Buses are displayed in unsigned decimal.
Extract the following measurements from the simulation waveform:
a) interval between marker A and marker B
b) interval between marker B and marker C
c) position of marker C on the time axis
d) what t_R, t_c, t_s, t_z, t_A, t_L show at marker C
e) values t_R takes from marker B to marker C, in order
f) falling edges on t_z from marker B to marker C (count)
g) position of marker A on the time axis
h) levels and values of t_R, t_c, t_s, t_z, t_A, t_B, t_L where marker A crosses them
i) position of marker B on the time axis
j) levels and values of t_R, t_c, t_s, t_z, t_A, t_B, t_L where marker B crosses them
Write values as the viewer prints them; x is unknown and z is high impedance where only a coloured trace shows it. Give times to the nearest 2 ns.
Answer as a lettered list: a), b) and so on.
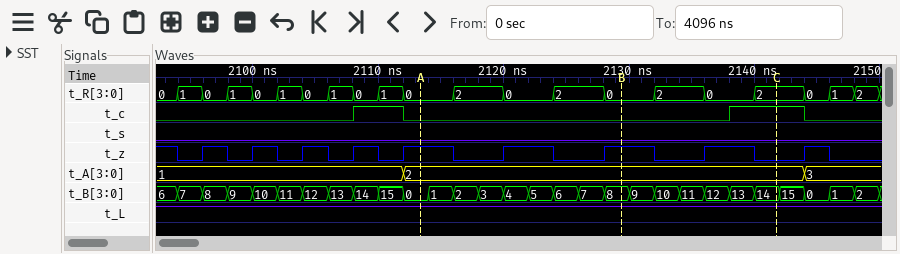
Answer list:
a) 16 ns
b) 12 ns
c) 2142 ns
d) t_R=2, t_c=1, t_s=0, t_z=0, t_A=2, t_L=1
e) 0, 2, 0, 2
f) 2
g) 2114 ns
h) t_R=0, t_c=0, t_s=0, t_z=1, t_A=2, t_B=0, t_L=1
i) 2130 ns
j) t_R=0, t_c=0, t_s=0, t_z=1, t_A=2, t_B=8, t_L=1
